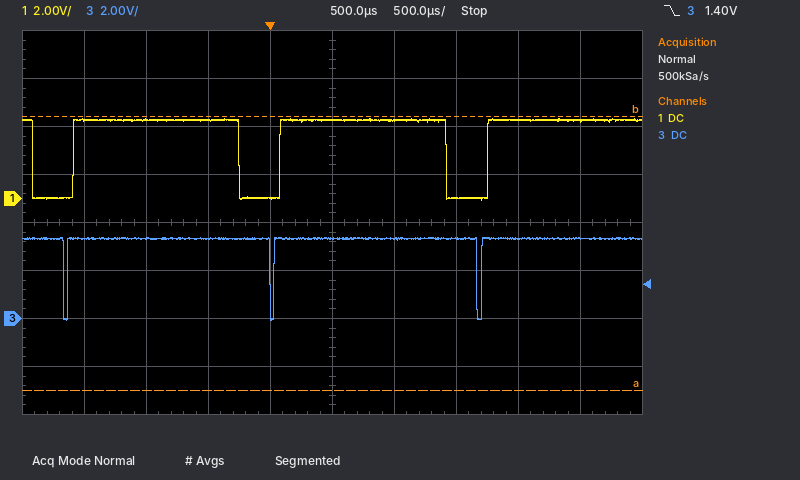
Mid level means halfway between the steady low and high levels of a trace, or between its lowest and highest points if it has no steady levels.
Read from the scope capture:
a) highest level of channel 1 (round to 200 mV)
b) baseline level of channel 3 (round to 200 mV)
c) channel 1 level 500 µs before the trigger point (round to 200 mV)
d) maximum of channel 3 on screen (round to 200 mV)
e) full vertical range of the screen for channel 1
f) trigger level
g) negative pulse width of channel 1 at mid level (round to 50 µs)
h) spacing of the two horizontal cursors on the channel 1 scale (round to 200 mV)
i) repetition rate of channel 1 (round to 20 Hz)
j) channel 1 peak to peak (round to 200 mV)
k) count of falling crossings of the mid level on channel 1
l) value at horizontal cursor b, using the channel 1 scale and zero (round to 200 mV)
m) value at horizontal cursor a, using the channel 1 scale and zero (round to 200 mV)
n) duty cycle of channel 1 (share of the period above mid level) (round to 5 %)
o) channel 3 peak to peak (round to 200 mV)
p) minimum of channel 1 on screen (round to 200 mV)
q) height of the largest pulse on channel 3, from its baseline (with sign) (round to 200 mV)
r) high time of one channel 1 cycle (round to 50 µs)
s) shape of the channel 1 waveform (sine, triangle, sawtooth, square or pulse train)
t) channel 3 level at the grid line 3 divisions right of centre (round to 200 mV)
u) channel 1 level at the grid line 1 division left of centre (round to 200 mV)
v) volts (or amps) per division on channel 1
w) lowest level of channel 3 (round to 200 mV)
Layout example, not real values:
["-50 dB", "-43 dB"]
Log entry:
["3.4 V", "3.4 V", "3.2 V", "3.4 V", "16 V", "1.40 V", "350 µs", "11.4 V", "600 Hz", "3.4 V", "3", "3.4 V", "-8.0 V", "80 %", "3.4 V", "0.0 V", "-3.4 V", "1.35 ms", "pulse train", "3.4 V", "0.0 V", "2 V", "0.0 V"]
